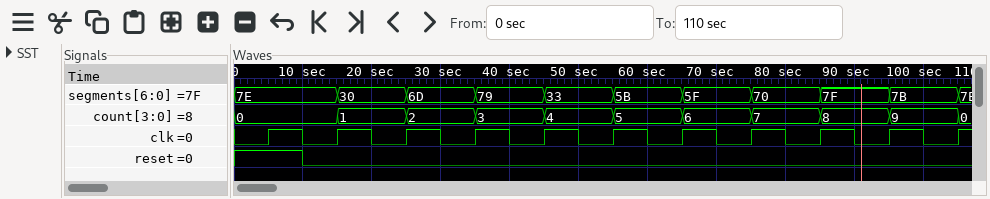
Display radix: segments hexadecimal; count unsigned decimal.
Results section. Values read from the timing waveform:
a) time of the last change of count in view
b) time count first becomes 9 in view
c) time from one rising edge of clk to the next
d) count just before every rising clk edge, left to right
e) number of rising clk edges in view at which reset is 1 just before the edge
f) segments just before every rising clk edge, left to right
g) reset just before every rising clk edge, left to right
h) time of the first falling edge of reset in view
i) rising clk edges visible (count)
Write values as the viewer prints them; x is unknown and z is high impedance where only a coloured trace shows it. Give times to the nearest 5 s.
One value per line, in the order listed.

105 s
95 s
10 s
0, 0, 1, 2, 3, 4, 5, 6, 7, 8, 9
1
7E, 7E, 30, 6D, 79, 33, 5B, 5F, 70, 7F, 7B
1 0 0 0 0 0 0 0 0 0 0
10 s
11
